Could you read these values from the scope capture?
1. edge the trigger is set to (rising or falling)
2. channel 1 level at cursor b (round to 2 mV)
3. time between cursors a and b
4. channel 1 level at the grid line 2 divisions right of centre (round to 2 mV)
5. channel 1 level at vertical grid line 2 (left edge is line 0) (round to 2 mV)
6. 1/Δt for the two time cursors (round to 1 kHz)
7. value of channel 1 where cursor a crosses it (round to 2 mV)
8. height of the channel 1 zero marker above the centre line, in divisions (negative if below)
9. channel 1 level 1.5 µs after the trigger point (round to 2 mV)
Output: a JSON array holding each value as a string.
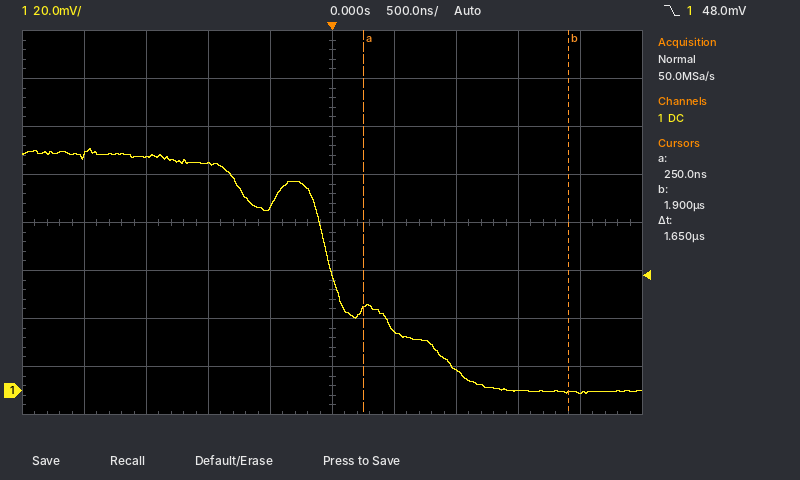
["falling", "0 mV", "1.65 µs", "8 mV", "98 mV", "606 kHz", "34 mV", "-3.5 div", "0 mV"]
